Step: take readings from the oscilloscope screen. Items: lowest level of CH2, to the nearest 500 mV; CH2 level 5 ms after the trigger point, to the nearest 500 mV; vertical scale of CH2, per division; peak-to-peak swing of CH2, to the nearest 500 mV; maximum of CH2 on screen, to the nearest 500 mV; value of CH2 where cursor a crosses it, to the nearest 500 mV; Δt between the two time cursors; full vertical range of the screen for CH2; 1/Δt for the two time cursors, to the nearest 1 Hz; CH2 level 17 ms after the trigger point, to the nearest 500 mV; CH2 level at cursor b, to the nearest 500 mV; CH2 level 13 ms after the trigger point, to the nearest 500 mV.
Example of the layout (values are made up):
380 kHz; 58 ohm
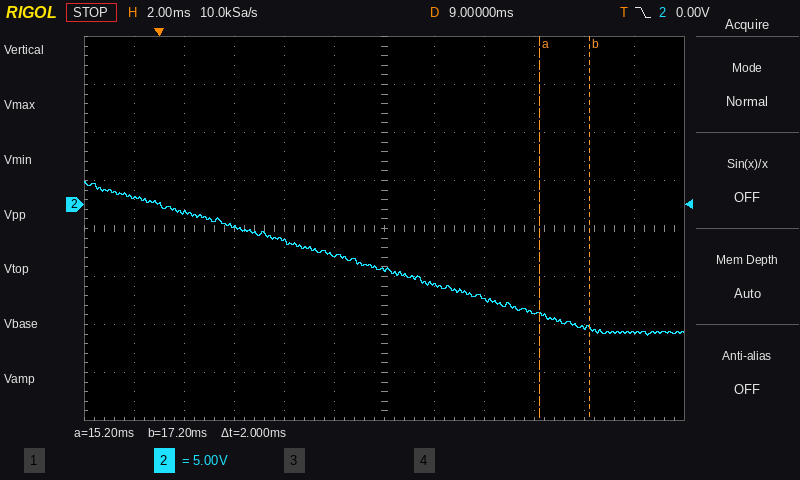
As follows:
-13.5 V; -4.0 V; 5 V; 16.0 V; 2.5 V; -11.5 V; 2 ms; 40 V; 500 Hz; -13.0 V; -13.0 V; -10.0 V
